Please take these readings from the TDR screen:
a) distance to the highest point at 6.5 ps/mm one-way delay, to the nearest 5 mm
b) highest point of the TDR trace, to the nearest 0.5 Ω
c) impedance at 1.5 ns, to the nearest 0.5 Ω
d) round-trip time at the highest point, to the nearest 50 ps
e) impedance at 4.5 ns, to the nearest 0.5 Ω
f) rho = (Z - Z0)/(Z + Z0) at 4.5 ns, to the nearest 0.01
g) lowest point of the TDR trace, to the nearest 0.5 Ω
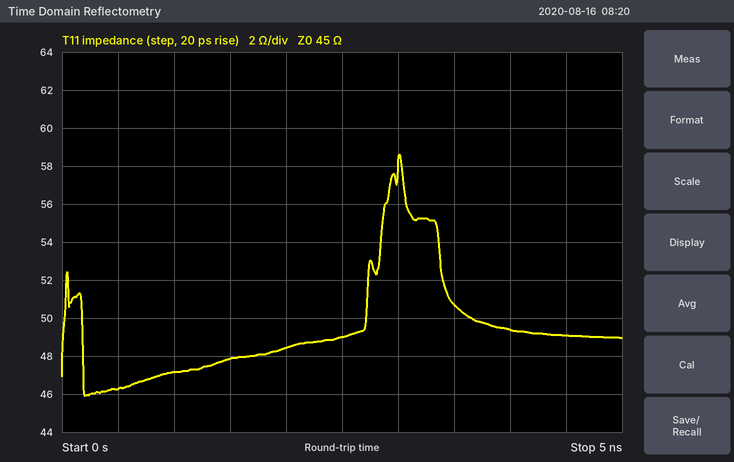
230 mm
58.5 Ω
48.0 Ω
3.00 ns
49.0 Ω
+0.04
46.0 Ω
